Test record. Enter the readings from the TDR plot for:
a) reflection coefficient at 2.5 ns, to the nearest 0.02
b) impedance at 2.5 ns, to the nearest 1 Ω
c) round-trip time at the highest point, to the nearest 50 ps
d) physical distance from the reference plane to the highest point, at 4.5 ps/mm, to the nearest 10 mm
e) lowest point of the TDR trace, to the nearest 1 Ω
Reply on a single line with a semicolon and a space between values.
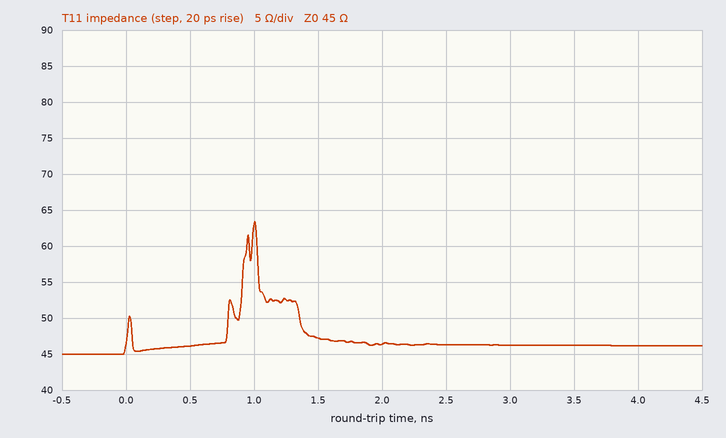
+0.02; 46 Ω; 1.00 ns; 110 mm; 45 Ω
